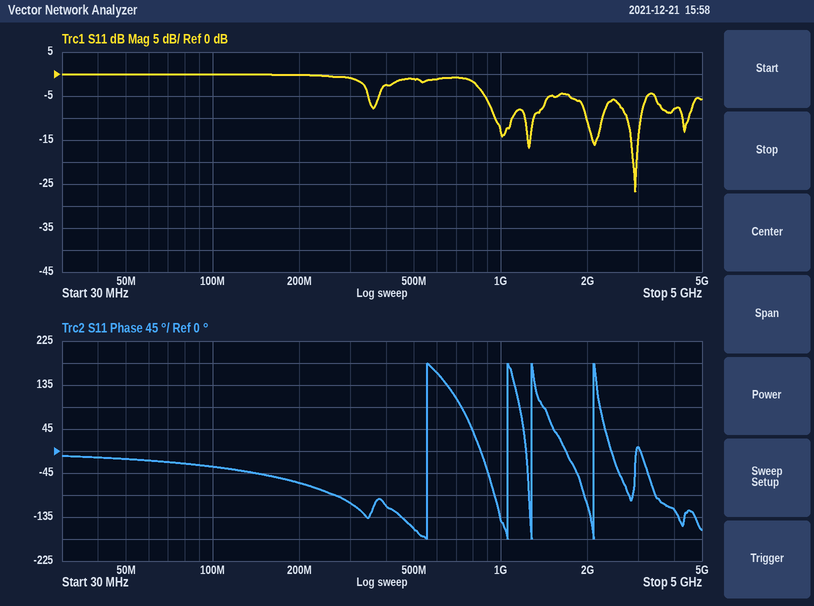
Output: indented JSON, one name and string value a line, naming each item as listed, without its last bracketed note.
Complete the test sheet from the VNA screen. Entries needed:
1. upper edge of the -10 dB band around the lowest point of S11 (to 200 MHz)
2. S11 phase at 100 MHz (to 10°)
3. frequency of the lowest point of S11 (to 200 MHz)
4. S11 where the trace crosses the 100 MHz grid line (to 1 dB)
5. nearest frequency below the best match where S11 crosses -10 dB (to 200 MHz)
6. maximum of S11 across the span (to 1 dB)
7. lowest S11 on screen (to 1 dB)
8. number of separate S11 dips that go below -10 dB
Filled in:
{
  "upper edge of the -10 dB band around the lowest point of S11": "3.0 GHz",
  "S11 phase at 100 MHz": "-30°",
  "frequency of the lowest point of S11": "3.0 GHz",
  "S11 where the trace crosses the 100 MHz grid line": "0 dB",
  "nearest frequency below the best match where S11 crosses -10 dB": "2.8 GHz",
  "maximum of S11 across the span": "0 dB",
  "lowest S11 on screen": "-27 dB",
  "number of separate S11 dips that go below -10 dB": "5"
}
